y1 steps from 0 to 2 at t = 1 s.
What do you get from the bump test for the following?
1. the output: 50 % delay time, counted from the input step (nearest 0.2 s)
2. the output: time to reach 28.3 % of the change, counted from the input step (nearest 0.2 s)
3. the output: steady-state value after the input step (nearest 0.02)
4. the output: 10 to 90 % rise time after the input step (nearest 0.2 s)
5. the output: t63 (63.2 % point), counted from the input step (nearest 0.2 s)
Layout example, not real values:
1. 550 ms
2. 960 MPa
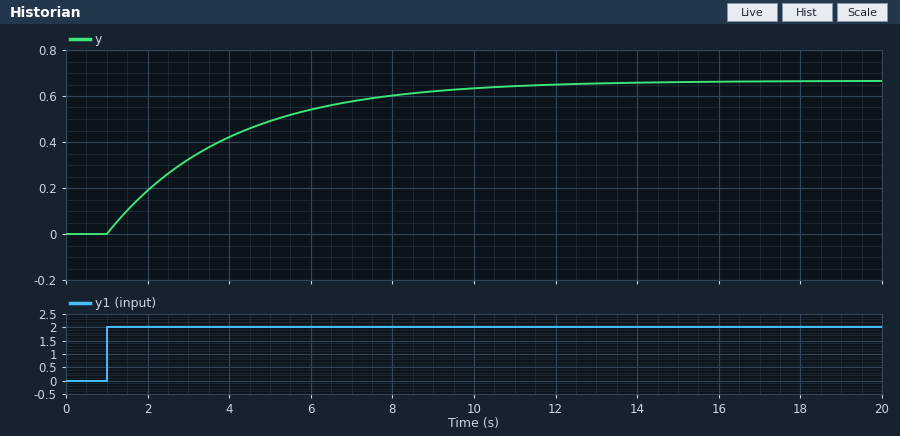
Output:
1. 2.0 s
2. 1.0 s
3. 0.66
4. 6.6 s
5. 3.0 s
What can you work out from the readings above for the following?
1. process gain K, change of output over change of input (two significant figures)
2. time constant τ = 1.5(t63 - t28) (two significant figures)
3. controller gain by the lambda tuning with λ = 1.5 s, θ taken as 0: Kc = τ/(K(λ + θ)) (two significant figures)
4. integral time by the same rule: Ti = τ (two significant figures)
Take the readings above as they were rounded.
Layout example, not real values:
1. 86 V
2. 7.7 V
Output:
1. 0.33
2. 3.0 s
3. 6.1
4. 3.0 s
